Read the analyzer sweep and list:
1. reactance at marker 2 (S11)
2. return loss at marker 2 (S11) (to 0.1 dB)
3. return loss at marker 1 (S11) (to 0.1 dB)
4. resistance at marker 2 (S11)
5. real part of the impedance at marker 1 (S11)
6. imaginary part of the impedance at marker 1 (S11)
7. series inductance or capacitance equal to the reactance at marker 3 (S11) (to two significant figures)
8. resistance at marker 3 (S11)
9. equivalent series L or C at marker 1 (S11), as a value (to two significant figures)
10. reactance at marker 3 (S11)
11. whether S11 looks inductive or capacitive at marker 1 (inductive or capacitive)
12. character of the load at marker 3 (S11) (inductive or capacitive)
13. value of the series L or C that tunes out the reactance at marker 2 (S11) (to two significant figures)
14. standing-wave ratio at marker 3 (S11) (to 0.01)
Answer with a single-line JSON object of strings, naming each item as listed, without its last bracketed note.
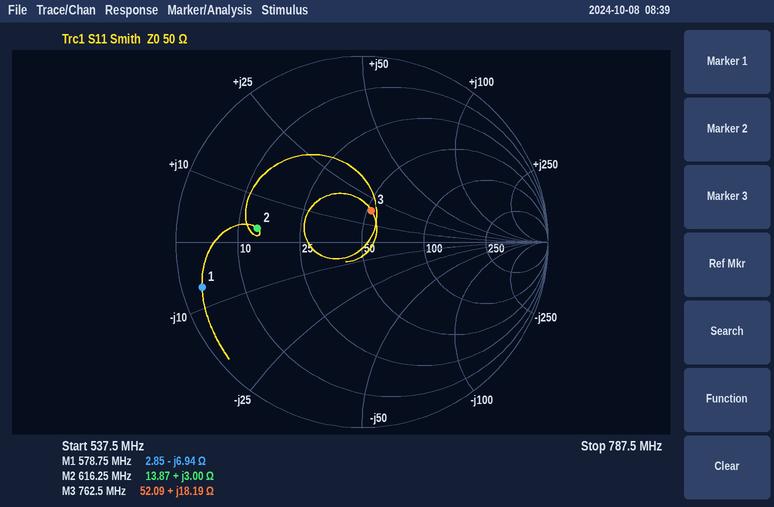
{"reactance at marker 2": "+3.00 Ω", "return loss at marker 2 (S11)": "4.9 dB", "return loss at marker 1 (S11)": "1.0 dB", "resistance at marker 2": "13.87 Ω", "real part of the impedance at marker 1": "2.85 Ω", "imaginary part of the impedance at marker 1": "-6.94 Ω", "series inductance or capacitance equal to the reactance at marker 3 (S11)": "3.8 nH", "resistance at marker 3": "52.09 Ω", "equivalent series L or C at marker 1 (S11), as a value": "40 pF", "reactance at marker 3": "+18.19 Ω", "whether S11 looks inductive or capacitive at marker 1": "capacitive", "character of the load at marker 3 (S11)": "inductive", "value of the series L or C that tunes out the reactance at marker 2 (S11)": "86 pF", "standing-wave ratio at marker 3 (S11)": "1.43"}
